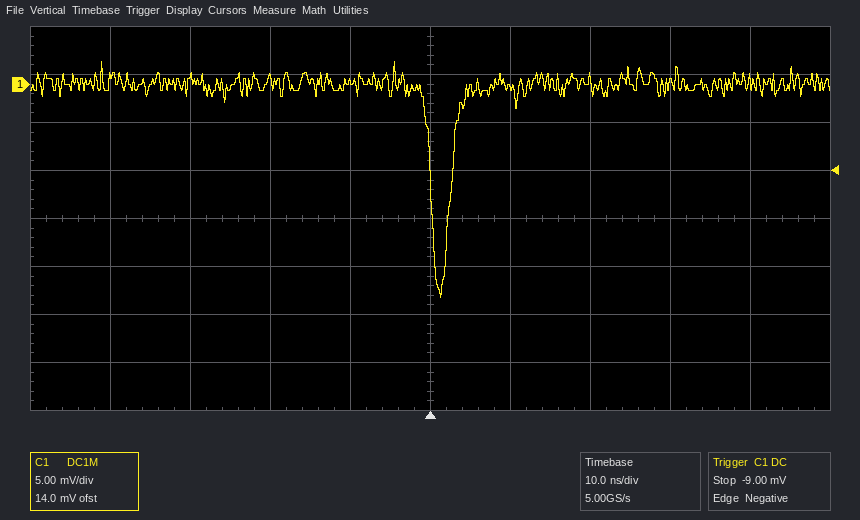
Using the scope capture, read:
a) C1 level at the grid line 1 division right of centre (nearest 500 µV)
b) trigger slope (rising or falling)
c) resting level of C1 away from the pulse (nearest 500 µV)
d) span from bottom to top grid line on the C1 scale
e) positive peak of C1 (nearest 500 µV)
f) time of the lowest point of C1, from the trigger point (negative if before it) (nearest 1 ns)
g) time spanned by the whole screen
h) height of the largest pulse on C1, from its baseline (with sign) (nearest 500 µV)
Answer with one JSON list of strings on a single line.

["-500 µV", "falling", "0.0 mV", "40 mV", "2.5 mV", "+1 ns", "100 ns", "-22.0 mV"]
